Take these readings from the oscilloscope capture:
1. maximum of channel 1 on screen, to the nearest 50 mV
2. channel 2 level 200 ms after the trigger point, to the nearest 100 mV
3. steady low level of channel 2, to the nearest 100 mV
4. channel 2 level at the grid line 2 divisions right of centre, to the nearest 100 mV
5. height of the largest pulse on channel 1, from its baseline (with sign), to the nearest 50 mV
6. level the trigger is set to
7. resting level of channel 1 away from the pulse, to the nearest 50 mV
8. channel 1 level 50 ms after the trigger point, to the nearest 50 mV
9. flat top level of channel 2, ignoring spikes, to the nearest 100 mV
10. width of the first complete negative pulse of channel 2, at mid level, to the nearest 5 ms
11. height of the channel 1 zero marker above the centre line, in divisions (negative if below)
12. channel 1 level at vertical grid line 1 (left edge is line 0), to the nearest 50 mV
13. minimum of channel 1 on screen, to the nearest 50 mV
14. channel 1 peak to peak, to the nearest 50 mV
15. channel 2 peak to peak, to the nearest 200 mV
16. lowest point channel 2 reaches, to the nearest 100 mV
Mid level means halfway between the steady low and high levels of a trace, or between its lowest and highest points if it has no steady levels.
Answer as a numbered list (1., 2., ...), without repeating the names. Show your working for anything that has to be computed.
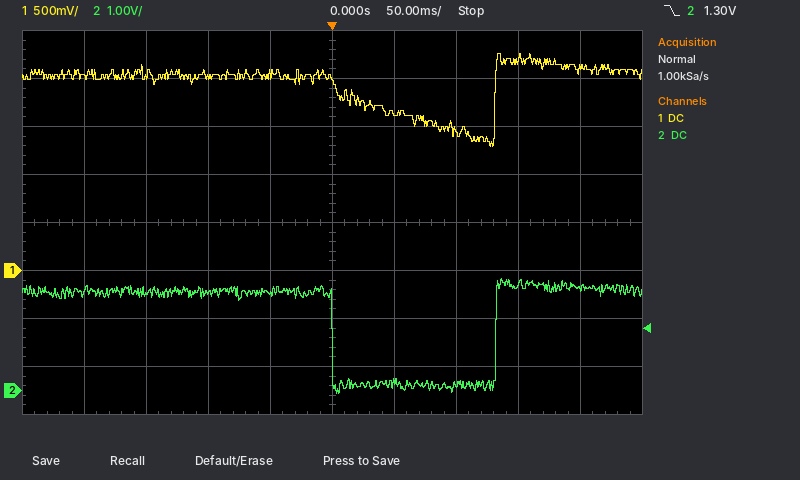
1. 2.25 V
2. 2.1 V
3. 100 mV
4. 100 mV
5. 1.30 V − (2.05 V) = -750 mV
6. 1.30 V
7. 2.05 V
8. 1.65 V
9. 2.1 V
10. 130 ms
11. -1.0 div
12. 2.00 V
13. 1.30 V
14. 2.25 V − (1.30 V) = 950 mV
15. 2.4 V
16. -100 mV
